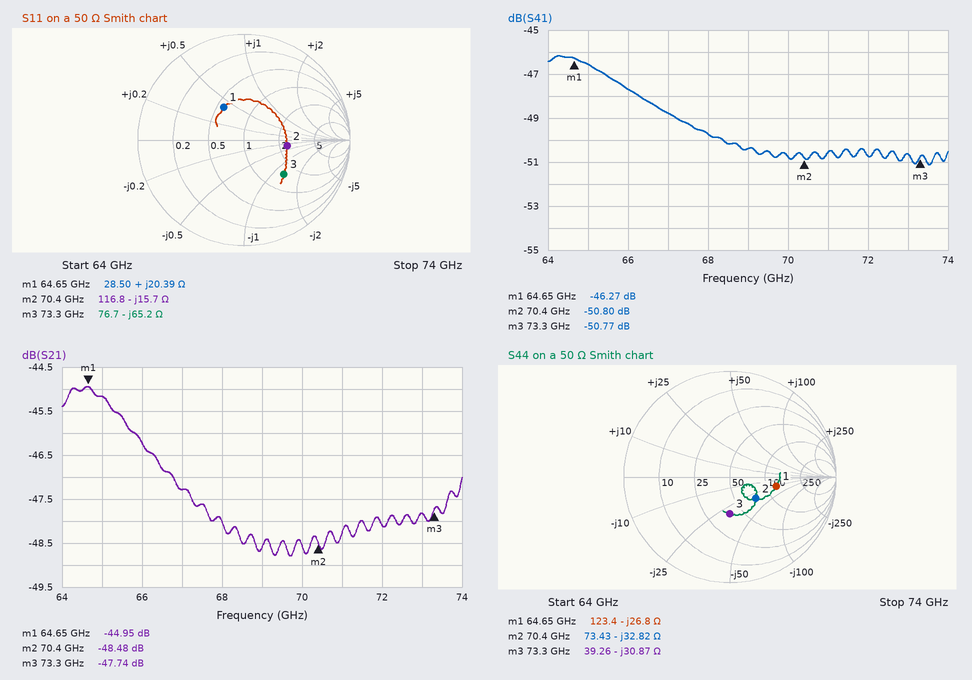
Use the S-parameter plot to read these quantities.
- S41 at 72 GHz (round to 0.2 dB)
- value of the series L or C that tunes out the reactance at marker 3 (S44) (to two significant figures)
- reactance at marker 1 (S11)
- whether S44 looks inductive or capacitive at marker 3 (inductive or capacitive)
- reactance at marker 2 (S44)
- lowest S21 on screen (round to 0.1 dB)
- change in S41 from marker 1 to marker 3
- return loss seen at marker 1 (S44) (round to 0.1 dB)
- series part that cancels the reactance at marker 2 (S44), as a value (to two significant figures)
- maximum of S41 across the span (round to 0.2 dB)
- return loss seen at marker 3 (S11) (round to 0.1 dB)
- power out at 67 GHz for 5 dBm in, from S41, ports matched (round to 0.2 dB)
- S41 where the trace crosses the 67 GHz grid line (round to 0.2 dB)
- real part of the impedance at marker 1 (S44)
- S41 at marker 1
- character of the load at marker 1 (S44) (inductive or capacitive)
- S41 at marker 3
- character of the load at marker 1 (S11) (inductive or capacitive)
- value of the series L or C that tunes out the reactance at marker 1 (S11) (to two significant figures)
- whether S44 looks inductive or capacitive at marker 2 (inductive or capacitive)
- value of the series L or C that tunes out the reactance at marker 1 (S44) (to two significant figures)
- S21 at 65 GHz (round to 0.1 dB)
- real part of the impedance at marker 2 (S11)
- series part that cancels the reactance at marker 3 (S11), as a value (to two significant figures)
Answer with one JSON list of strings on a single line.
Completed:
["-50.8 dB", "67 pH", "+20.39 Ω", "capacitive", "-32.82 Ω", "-48.8 dB", "-4.50 dB", "7.0 dB", "74 pH", "-46.2 dB", "6.1 dB", "-43.8 dBm", "-48.8 dB", "123.4 Ω", "-46.27 dB", "capacitive", "-50.77 dB", "inductive", "120 fF", "capacitive", "66 pH", "-45.2 dB", "116.8 Ω", "140 pH"]
